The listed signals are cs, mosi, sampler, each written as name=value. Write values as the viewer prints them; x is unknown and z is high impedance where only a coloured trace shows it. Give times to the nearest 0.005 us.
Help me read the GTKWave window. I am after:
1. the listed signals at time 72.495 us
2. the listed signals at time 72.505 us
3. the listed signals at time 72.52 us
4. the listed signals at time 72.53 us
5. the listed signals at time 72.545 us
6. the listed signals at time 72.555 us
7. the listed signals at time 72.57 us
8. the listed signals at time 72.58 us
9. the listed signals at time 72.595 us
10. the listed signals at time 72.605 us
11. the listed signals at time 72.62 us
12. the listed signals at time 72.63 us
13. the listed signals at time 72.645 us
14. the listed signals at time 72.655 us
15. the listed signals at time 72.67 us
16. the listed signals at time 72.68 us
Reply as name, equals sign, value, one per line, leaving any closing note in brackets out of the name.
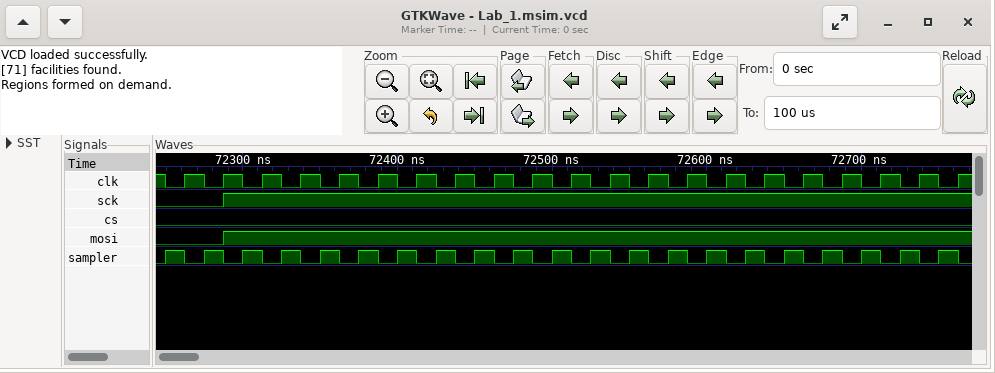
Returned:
the listed signals at time 72.495 us = cs=0, mosi=1, sampler=0
the listed signals at time 72.505 us = cs=0, mosi=1, sampler=1
the listed signals at time 72.52 us = cs=0, mosi=1, sampler=0
the listed signals at time 72.53 us = cs=0, mosi=1, sampler=1
the listed signals at time 72.545 us = cs=0, mosi=1, sampler=0
the listed signals at time 72.555 us = cs=0, mosi=1, sampler=1
the listed signals at time 72.57 us = cs=0, mosi=1, sampler=0
the listed signals at time 72.58 us = cs=0, mosi=1, sampler=1
the listed signals at time 72.595 us = cs=0, mosi=1, sampler=0
the listed signals at time 72.605 us = cs=0, mosi=1, sampler=1
the listed signals at time 72.62 us = cs=0, mosi=1, sampler=0
the listed signals at time 72.63 us = cs=0, mosi=1, sampler=1
the listed signals at time 72.645 us = cs=0, mosi=1, sampler=0
the listed signals at time 72.655 us = cs=0, mosi=1, sampler=1
the listed signals at time 72.67 us = cs=0, mosi=1, sampler=0
the listed signals at time 72.68 us = cs=0, mosi=1, sampler=1
